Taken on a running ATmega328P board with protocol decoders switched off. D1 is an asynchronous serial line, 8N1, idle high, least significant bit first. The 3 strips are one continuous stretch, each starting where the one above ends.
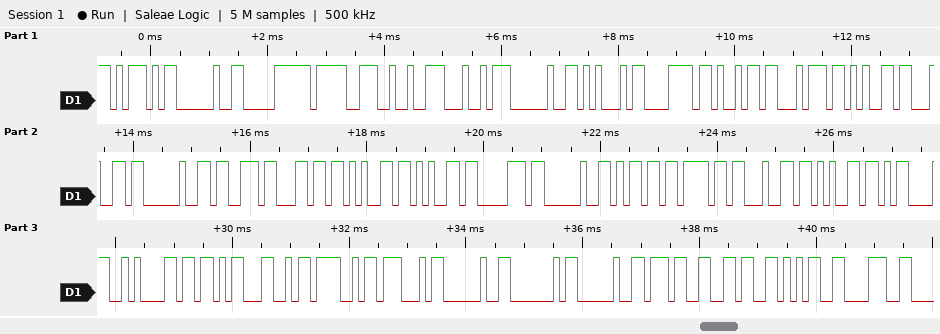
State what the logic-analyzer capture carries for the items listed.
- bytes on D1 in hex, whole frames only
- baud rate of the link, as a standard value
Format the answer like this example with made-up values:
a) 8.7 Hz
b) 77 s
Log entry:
a) 5D 20 F0 9F 92 A4 20 45 78 69 74 65 64 20 73 6C 65 65 70 20 6D 6F 64 65 0D 0A 5B 4C 4F 47 20 40 20 37 36 35 38
b) 9600 baud
